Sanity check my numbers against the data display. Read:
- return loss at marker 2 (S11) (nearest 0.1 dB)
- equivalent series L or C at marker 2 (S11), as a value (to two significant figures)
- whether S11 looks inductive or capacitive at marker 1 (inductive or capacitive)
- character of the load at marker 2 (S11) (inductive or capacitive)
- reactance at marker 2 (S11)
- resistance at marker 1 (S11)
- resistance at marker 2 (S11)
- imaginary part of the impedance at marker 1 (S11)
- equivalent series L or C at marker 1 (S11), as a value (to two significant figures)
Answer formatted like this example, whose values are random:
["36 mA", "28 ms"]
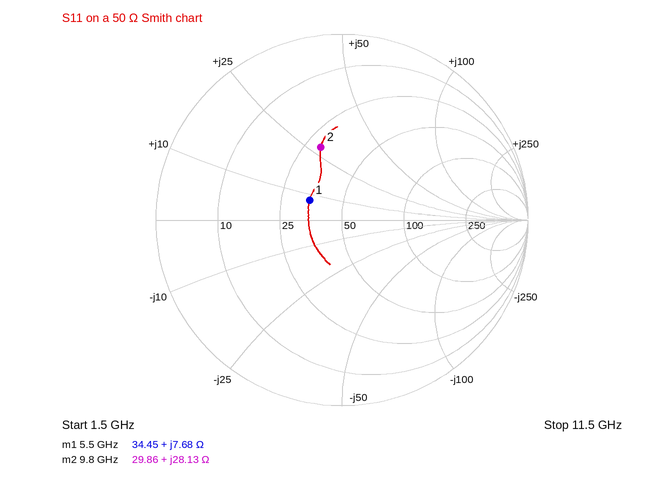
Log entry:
["7.8 dB", "460 pH", "inductive", "inductive", "+28.13 Ω", "34.45 Ω", "29.86 Ω", "+7.68 Ω", "220 pH"]
